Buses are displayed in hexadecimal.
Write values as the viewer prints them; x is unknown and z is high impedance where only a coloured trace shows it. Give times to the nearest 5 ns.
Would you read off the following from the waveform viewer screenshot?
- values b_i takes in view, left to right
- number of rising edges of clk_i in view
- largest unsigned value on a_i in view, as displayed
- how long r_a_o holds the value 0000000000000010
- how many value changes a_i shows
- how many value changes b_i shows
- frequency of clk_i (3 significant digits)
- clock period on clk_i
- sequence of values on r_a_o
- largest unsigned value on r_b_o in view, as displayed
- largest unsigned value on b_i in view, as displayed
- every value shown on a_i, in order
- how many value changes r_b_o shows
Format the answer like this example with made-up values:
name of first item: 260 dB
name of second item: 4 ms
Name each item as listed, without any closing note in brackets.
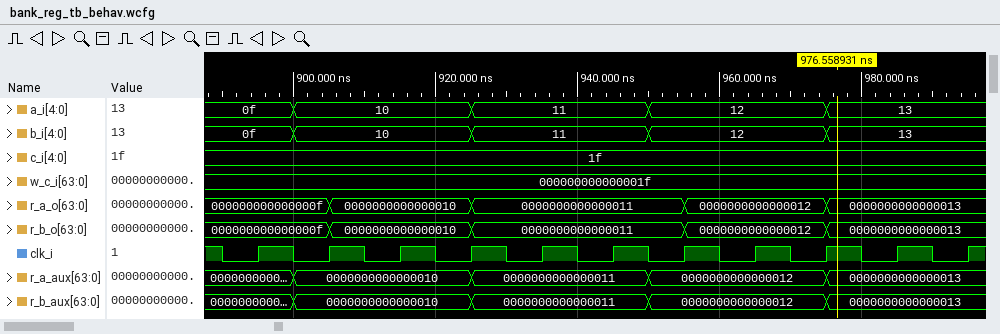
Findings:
values b_i takes in view, left to right: 0f, 10, 11, 12, 13
number of rising edges of clk_i in view: 11
largest unsigned value on a_i in view, as displayed: 13
how long r_a_o holds the value 0000000000000010: 20 ns
how many value changes a_i shows: 4
how many value changes b_i shows: 4
frequency of clk_i: 100 MHz
clock period on clk_i: 10 ns
sequence of values on r_a_o: 000000000000000f, 0000000000000010, 0000000000000011, 0000000000000012, 0000000000000013
largest unsigned value on r_b_o in view, as displayed: 0000000000000013
largest unsigned value on b_i in view, as displayed: 13
every value shown on a_i, in order: 0f, 10, 11, 12, 13
how many value changes r_b_o shows: 4
